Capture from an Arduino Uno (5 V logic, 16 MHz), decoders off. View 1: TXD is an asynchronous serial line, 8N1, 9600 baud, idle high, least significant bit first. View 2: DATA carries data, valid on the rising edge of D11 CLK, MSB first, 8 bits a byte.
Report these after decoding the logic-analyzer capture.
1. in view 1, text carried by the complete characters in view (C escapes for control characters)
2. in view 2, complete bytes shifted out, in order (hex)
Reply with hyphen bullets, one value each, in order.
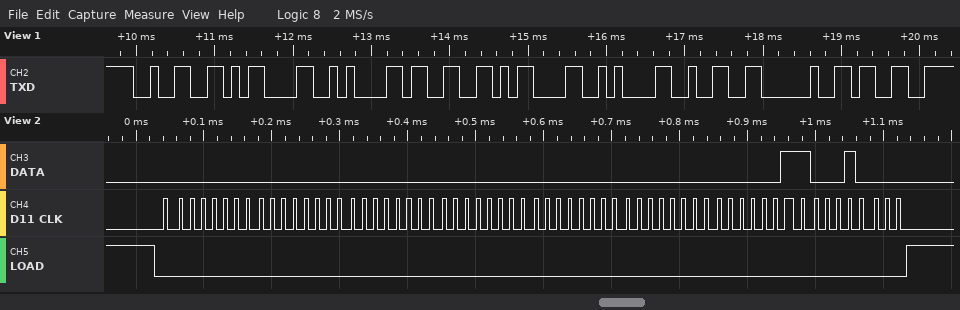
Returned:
- "2\r\n3\r\n2 3"
- 00 00 00 00 00 00 03 10
